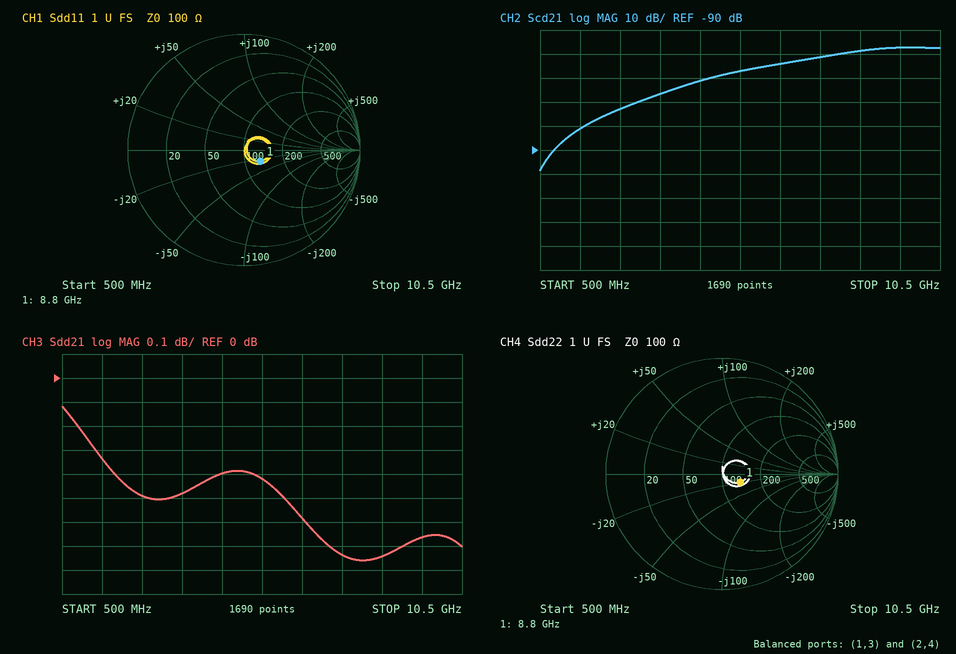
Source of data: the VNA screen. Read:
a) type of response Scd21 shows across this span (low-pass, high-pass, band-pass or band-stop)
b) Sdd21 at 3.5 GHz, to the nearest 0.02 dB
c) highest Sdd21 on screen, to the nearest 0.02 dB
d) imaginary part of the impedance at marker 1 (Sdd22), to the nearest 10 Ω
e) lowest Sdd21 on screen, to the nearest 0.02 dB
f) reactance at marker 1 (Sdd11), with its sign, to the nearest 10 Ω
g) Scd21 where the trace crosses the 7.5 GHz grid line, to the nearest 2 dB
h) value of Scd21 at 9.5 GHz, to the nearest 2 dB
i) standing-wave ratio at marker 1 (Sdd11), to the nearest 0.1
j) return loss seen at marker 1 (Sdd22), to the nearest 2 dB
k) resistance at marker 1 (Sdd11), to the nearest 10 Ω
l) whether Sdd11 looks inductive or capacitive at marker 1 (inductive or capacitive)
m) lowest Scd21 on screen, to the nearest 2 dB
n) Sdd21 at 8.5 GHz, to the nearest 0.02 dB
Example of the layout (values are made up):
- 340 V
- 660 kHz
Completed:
- high-pass
- -0.48 dB
- -0.12 dB
- -20 Ω
- -0.76 dB
- -30 Ω
- -52 dB
- -48 dB
- 1.4
- 16 dB
- 130 Ω
- capacitive
- -98 dB
- -0.74 dB
